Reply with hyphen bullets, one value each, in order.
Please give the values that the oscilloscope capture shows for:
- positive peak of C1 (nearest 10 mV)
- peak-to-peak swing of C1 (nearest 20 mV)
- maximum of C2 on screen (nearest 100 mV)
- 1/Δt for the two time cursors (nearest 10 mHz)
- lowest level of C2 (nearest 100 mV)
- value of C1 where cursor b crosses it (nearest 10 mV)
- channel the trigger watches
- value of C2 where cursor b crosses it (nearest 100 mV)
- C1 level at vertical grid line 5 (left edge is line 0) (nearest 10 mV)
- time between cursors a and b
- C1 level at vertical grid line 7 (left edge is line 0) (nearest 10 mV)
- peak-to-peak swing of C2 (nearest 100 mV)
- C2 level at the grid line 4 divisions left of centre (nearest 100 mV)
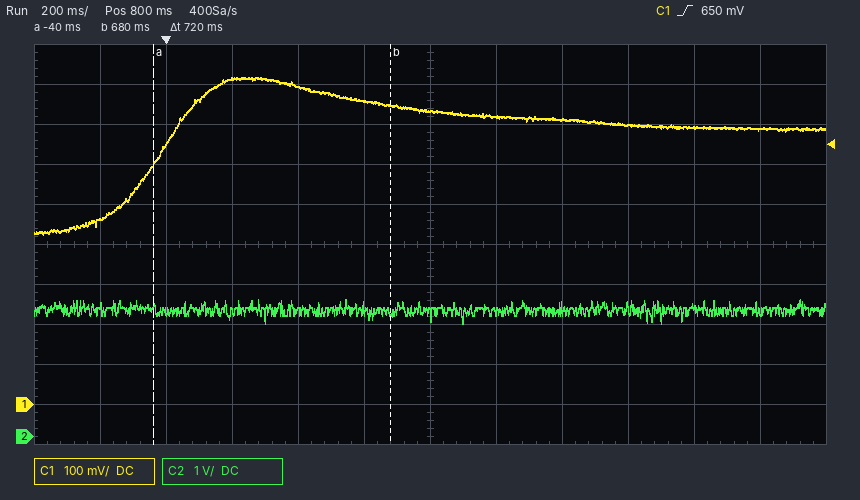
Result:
- 820 mV
- 400 mV
- 3.4 V
- 1.39 Hz
- 2.8 V
- 750 mV
- C1
- 3.1 V
- 760 mV
- 720 ms
- 720 mV
- 600 mV
- 3.1 V
